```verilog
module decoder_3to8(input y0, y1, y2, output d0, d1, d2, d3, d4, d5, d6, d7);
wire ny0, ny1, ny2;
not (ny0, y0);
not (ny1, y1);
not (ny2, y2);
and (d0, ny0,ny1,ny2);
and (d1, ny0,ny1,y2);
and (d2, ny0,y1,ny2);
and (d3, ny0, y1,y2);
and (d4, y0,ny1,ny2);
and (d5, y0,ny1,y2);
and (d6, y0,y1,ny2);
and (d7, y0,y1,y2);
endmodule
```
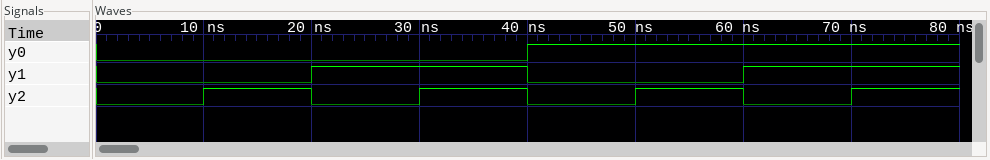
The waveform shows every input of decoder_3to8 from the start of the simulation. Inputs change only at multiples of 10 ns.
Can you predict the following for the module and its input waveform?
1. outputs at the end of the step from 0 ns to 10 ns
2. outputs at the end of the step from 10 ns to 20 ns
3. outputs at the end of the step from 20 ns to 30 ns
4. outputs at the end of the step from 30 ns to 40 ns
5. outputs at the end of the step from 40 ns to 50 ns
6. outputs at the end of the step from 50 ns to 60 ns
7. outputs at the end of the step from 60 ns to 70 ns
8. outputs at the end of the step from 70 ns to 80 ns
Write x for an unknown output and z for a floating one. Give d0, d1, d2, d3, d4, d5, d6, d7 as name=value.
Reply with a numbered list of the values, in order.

1. d0=1, d1=0, d2=0, d3=0, d4=0, d5=0, d6=0, d7=0
2. d0=0, d1=1, d2=0, d3=0, d4=0, d5=0, d6=0, d7=0
3. d0=0, d1=0, d2=1, d3=0, d4=0, d5=0, d6=0, d7=0
4. d0=0, d1=0, d2=0, d3=1, d4=0, d5=0, d6=0, d7=0
5. d0=0, d1=0, d2=0, d3=0, d4=1, d5=0, d6=0, d7=0
6. d0=0, d1=0, d2=0, d3=0, d4=0, d5=1, d6=0, d7=0
7. d0=0, d1=0, d2=0, d3=0, d4=0, d5=0, d6=1, d7=0
8. d0=0, d1=0, d2=0, d3=0, d4=0, d5=0, d6=0, d7=1
